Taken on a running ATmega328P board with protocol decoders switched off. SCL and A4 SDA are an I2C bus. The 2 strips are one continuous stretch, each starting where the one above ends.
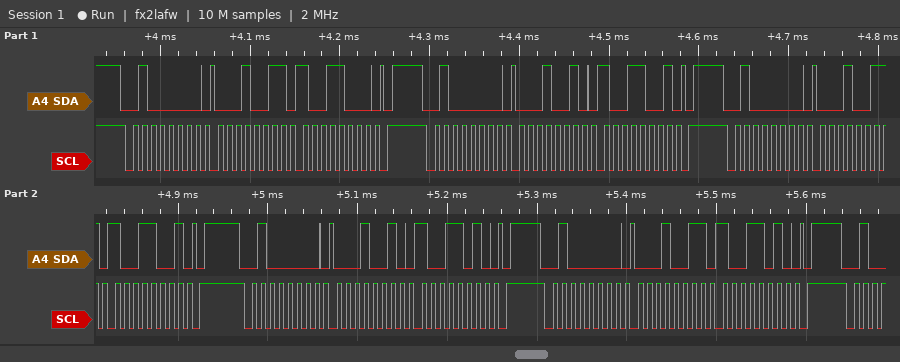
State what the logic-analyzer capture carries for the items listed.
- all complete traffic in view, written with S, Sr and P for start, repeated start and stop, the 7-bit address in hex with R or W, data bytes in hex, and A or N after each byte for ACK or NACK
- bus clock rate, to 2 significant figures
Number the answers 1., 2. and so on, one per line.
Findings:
1. S 20W A 13 A 98 A P S 20W A 12 A 99 A P S 20W A 13 A 99 A P S 20W A 12 A 9A A P S 20W A 13 A 9A A P
2. 100 kHz
